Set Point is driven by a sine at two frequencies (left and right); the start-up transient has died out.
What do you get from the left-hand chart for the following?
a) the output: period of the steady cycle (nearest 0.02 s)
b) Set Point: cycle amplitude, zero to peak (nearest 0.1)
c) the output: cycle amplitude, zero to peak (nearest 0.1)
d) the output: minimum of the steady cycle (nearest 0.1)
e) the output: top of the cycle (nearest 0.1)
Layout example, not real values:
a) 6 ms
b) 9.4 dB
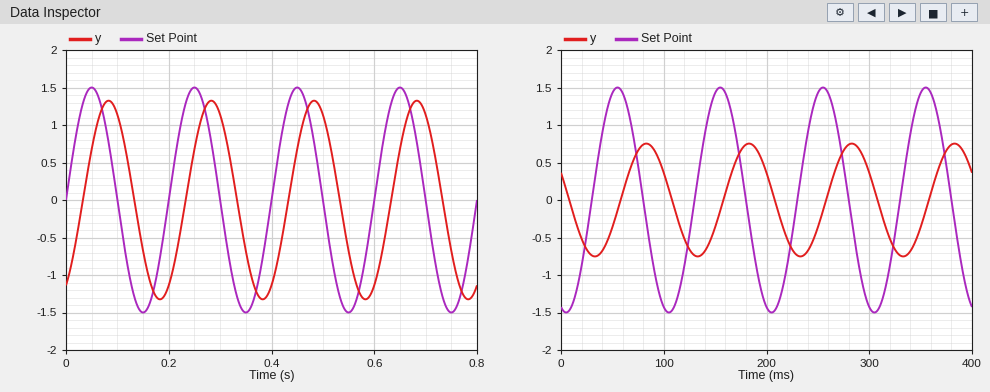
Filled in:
a) 0.20 s
b) 1.5
c) 1.3
d) -1.3
e) 1.3
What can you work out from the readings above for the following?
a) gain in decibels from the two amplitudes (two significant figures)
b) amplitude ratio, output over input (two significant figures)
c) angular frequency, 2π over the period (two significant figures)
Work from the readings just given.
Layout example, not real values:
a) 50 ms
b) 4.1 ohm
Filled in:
a) -1.2 dB
b) 0.87
c) 31 rad/s
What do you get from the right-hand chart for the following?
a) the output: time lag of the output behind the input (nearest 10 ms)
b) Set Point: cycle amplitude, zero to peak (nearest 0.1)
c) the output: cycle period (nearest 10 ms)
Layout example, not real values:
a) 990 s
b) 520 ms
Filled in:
a) 30 ms
b) 1.5
c) 100 ms
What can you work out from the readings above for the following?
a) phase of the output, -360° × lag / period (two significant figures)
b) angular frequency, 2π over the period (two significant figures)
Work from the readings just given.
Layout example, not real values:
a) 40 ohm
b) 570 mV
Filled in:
a) -110°
b) 0.063 rad/ms
